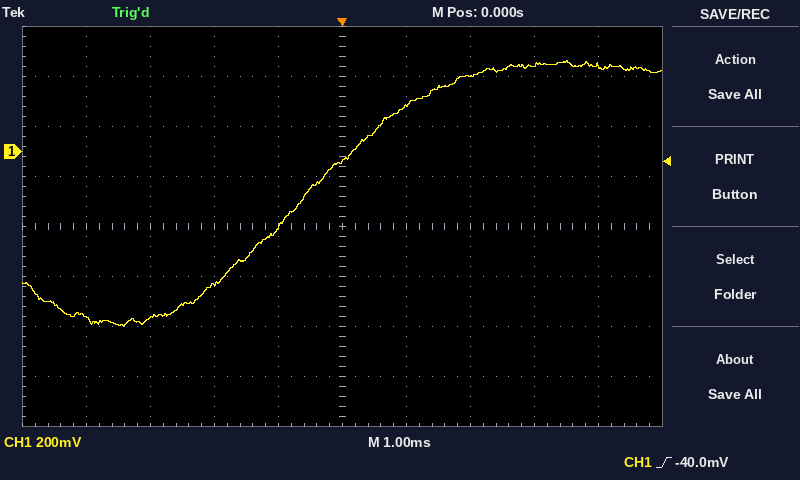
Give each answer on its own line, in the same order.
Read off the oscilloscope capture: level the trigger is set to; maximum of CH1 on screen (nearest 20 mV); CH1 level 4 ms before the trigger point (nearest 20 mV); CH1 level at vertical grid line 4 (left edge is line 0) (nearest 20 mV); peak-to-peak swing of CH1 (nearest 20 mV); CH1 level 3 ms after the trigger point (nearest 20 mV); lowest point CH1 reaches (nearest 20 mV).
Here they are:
-40.0 mV
360 mV
-660 mV
-300 mV
1.06 V
340 mV
-700 mV
